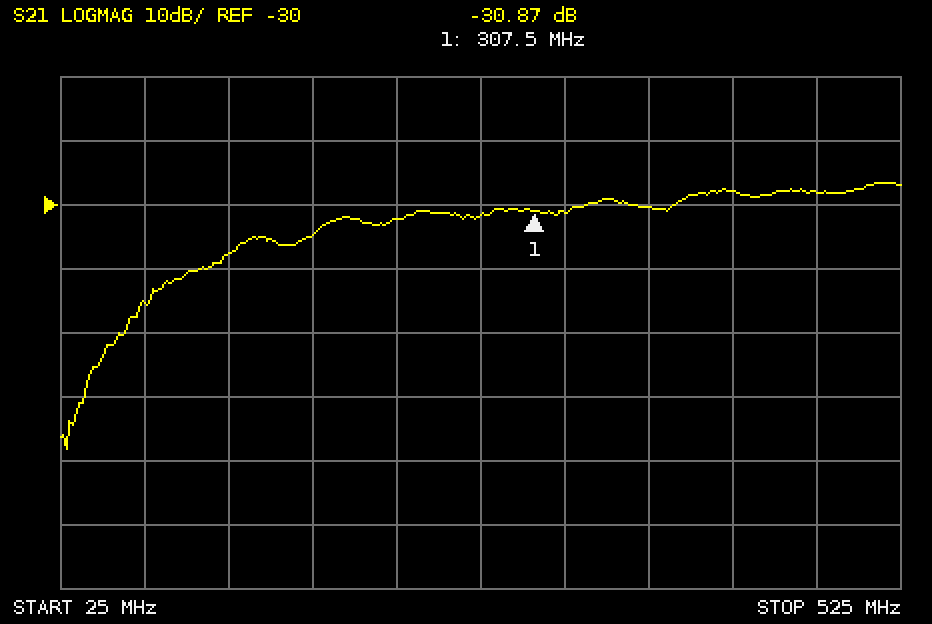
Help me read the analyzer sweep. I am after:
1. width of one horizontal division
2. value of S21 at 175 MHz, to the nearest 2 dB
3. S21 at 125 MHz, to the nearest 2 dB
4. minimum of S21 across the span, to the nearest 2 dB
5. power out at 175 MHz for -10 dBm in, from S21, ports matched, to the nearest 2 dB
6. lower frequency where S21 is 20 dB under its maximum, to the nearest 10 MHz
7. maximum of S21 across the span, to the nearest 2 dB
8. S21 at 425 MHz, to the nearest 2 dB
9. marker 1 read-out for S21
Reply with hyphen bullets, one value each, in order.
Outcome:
- 50 MHz
- -34 dB
- -38 dB
- -68 dB
- -44 dBm
- 70 MHz
- -26 dB
- -28 dB
- -30.87 dB
